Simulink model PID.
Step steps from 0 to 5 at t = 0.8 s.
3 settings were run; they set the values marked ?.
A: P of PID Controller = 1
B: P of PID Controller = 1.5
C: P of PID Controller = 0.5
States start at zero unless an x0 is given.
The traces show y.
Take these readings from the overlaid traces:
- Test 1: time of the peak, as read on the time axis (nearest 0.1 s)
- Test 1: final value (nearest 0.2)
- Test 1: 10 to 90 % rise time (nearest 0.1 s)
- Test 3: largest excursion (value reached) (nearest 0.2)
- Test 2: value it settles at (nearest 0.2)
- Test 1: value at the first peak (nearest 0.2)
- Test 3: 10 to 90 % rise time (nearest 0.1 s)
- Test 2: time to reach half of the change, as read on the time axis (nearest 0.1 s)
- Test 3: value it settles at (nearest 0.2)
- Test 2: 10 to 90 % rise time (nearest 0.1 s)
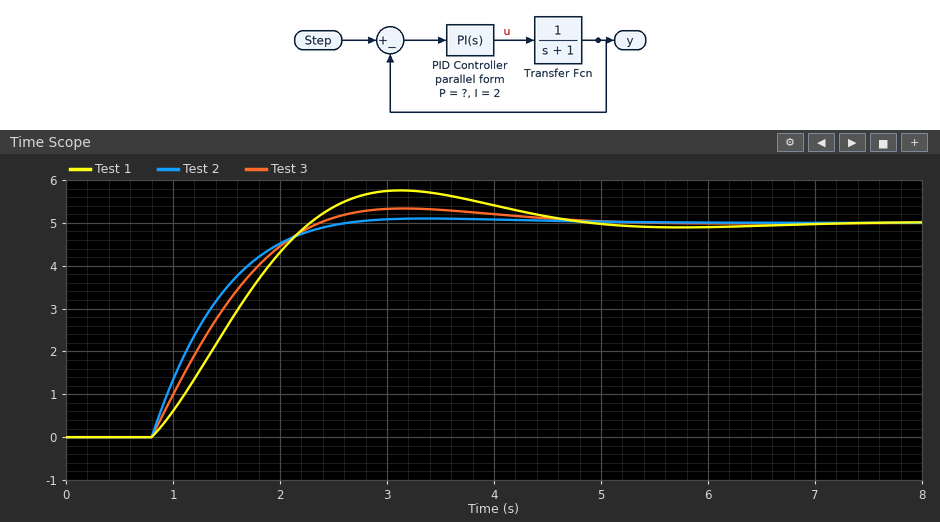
3.1 s
5.0
1.1 s
5.4
5.0
5.8
1.1 s
1.2 s
5.0
1.1 s
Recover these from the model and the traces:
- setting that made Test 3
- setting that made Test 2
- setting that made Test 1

A
B
C
